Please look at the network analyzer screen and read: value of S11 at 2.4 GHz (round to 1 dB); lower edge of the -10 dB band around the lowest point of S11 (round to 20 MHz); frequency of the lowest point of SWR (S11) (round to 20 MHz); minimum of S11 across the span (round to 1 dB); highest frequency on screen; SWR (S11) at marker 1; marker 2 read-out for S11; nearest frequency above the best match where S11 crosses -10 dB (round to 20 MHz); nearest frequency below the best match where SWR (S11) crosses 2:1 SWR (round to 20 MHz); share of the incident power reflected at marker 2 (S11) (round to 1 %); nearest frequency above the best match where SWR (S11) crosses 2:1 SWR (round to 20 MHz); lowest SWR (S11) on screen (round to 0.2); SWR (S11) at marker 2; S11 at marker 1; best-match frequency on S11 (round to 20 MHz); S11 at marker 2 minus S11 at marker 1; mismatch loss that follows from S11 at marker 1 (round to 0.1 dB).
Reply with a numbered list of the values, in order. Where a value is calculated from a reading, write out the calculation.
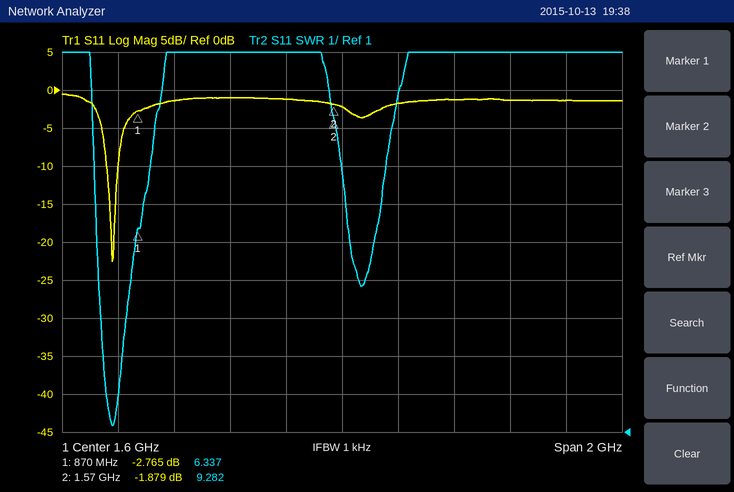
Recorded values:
1. -1 dB
2. 760 MHz
3. 780 MHz
4. -23 dB
5. 2.6 GHz
6. 6.337
7. -1.879 dB
8. 800 MHz
9. 760 MHz
10. 10^(-1.879/10) ≈ 65 %
11. 800 MHz
12. 1.2
13. 9.282
14. -2.765 dB
15. 780 MHz
16. -1.879 − (-2.765) = 0.886 dB
17. −10 log10(1 − 10^(-2.765/10)) ≈ 3.3 dB
